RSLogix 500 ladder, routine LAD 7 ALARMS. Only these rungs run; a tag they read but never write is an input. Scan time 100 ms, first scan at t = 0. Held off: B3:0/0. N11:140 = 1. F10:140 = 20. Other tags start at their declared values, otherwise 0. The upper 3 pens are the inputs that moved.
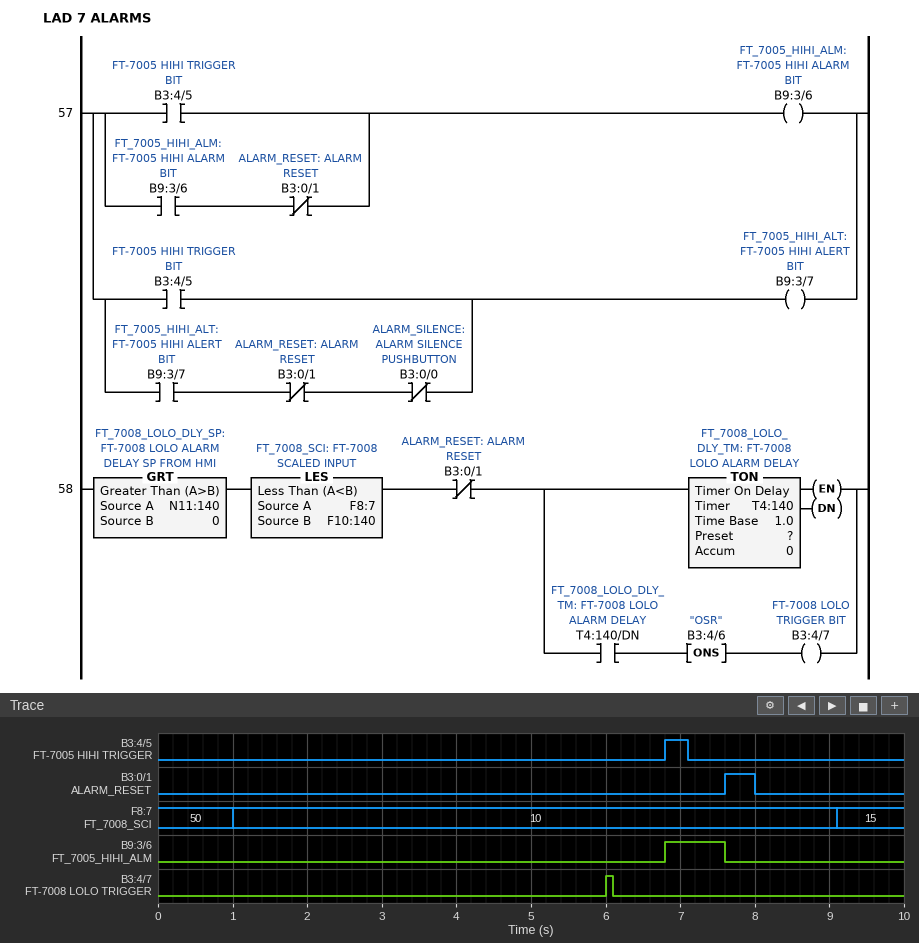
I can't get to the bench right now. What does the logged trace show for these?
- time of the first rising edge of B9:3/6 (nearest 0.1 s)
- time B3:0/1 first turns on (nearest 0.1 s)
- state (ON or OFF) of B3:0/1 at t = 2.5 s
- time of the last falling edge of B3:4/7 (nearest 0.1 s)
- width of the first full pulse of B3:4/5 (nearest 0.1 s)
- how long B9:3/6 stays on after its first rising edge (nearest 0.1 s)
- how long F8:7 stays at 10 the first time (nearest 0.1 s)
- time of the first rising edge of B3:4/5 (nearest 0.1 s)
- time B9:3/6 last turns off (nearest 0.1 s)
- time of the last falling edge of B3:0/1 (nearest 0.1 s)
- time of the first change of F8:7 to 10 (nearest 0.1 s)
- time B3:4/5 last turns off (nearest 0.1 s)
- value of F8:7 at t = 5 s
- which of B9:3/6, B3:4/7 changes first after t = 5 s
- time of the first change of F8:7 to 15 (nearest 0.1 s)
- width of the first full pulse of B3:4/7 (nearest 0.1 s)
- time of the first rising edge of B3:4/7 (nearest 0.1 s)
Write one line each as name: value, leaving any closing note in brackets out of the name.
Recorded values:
time of the first rising edge of B9:3/6: 6.8 s
time B3:0/1 first turns on: 7.6 s
state (ON or OFF) of B3:0/1 at t = 2.5 s: OFF
time of the last falling edge of B3:4/7: 6.1 s
width of the first full pulse of B3:4/5: 0.3 s
how long B9:3/6 stays on after its first rising edge: 0.8 s
how long F8:7 stays at 10 the first time: 8.1 s
time of the first rising edge of B3:4/5: 6.8 s
time B9:3/6 last turns off: 7.6 s
time of the last falling edge of B3:0/1: 8.0 s
time of the first change of F8:7 to 10: 1.0 s
time B3:4/5 last turns off: 7.1 s
value of F8:7 at t = 5 s: 10
which of B9:3/6, B3:4/7 changes first after t = 5 s: B3:4/7
time of the first change of F8:7 to 15: 9.1 s
width of the first full pulse of B3:4/7: 0.1 s
time of the first rising edge of B3:4/7: 6.0 s
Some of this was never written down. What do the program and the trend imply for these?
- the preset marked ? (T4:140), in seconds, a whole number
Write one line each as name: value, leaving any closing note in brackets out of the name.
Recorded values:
the preset marked ? (T4:140), in seconds, a whole number: 5 s
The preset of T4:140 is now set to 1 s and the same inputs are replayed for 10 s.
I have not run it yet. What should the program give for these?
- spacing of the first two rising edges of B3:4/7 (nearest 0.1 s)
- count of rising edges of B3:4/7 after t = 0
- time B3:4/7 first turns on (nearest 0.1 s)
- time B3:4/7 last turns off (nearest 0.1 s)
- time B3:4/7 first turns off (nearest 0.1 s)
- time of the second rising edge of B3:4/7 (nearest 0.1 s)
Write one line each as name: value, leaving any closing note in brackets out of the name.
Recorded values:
spacing of the first two rising edges of B3:4/7: 7.0 s
count of rising edges of B3:4/7 after t = 0: 2
time B3:4/7 first turns on: 2.0 s
time B3:4/7 last turns off: 9.1 s
time B3:4/7 first turns off: 2.1 s
time of the second rising edge of B3:4/7: 9.0 s
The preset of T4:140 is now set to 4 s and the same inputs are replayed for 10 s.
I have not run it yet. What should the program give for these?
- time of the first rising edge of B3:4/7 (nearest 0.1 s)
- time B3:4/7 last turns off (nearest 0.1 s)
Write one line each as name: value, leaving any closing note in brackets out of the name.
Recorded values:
time of the first rising edge of B3:4/7: 5.0 s
time B3:4/7 last turns off: 5.1 s
